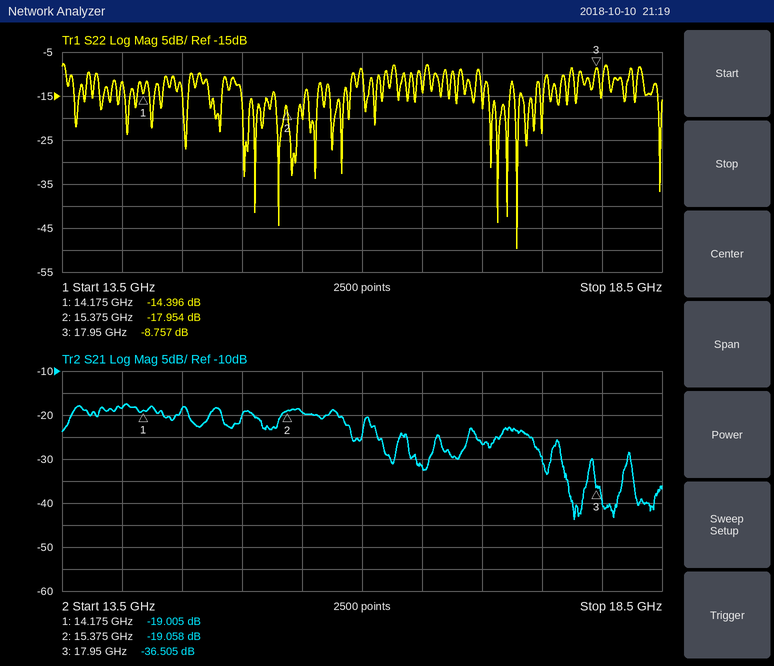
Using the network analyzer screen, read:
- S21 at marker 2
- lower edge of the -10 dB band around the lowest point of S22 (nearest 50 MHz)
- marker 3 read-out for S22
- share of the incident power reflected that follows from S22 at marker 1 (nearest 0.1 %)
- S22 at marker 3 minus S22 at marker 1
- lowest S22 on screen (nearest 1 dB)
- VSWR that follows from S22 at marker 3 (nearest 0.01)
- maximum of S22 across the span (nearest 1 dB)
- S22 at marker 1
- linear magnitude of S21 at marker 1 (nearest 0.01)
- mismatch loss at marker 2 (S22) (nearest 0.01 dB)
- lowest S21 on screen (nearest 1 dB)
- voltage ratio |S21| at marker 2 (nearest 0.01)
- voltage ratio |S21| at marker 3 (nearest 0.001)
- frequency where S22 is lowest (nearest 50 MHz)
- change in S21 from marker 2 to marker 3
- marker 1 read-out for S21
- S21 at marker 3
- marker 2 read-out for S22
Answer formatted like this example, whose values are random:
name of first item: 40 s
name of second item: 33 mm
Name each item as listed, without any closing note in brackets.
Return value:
S21 at marker 2: -19.058 dB
lower edge of the -10 dB band around the lowest point of S22: 17.00 GHz
marker 3 read-out for S22: -8.757 dB
share of the incident power reflected that follows from S22 at marker 1: 3.6 %
S22 at marker 3 minus S22 at marker 1: 5.639 dB
lowest S22 on screen: -50 dB
VSWR that follows from S22 at marker 3: 2.15
maximum of S22 across the span: -8 dB
S22 at marker 1: -14.396 dB
linear magnitude of S21 at marker 1: 0.11
mismatch loss at marker 2 (S22): 0.07 dB
lowest S21 on screen: -44 dB
voltage ratio |S21| at marker 2: 0.11
voltage ratio |S21| at marker 3: 0.015
frequency where S22 is lowest: 17.30 GHz
change in S21 from marker 2 to marker 3: -17.447 dB
marker 1 read-out for S21: -19.005 dB
S21 at marker 3: -36.505 dB
marker 2 read-out for S22: -17.954 dB
